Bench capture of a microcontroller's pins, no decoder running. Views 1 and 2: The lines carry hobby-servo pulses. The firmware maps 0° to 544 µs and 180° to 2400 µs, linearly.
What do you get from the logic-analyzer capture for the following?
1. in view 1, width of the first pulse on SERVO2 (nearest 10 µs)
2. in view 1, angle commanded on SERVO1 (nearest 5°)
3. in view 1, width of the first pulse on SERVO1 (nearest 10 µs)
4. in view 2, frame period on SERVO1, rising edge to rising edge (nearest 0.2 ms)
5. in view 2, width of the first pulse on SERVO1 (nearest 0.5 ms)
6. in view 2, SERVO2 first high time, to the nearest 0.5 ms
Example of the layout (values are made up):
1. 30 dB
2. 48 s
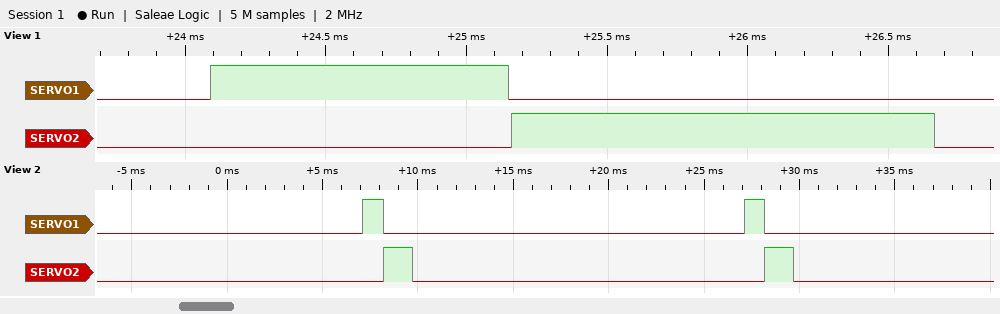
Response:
1. 1500 µs
2. 50°
3. 1060 µs
4. 20.0 ms
5. 1.0 ms
6. 1.5 ms
